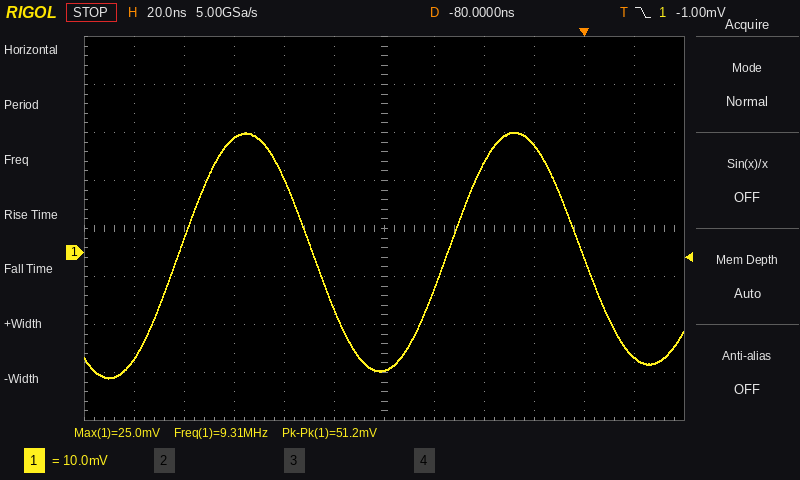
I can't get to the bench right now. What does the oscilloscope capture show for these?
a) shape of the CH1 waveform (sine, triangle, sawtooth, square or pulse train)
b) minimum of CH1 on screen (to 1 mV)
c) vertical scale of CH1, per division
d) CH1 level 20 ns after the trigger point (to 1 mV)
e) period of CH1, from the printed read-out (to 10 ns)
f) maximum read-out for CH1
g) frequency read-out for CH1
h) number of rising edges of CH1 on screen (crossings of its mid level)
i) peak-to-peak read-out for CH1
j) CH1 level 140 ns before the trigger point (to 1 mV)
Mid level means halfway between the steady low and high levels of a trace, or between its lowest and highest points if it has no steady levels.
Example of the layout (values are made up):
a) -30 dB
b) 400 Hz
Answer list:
a) sine
b) -26 mV
c) 10 mV
d) -22 mV
e) 110 ns
f) 25.0 mV
g) 9.31 MHz
h) 2
i) 51.2 mV
j) 24 mV
